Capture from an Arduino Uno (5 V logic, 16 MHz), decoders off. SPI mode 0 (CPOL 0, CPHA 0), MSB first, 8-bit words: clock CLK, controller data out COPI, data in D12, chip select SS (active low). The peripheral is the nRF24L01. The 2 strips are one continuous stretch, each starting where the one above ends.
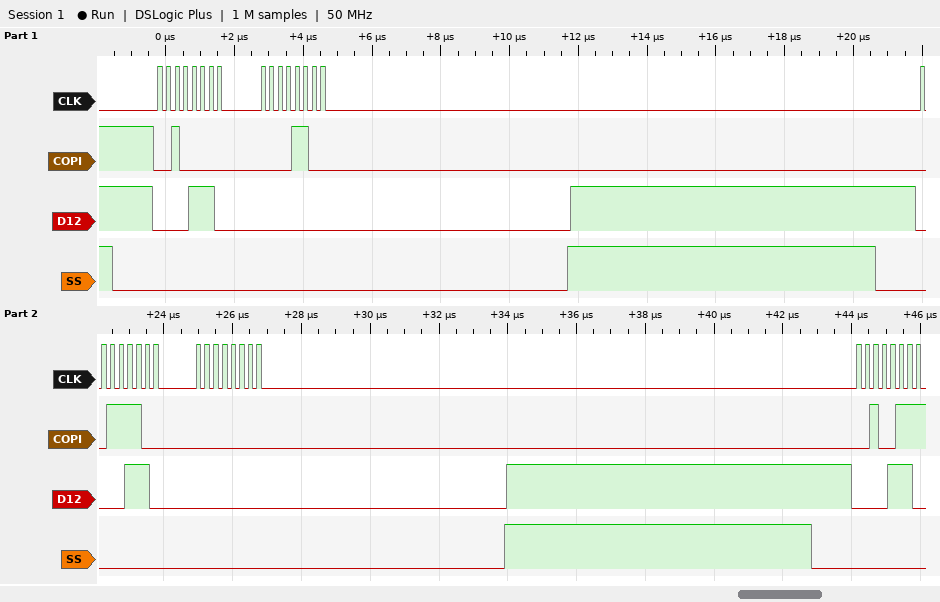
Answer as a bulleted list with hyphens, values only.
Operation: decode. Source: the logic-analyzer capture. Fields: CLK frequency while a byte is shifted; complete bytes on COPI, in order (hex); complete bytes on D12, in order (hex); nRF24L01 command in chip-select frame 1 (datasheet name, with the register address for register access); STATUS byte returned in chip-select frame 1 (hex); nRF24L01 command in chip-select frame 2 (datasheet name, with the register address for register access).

- 4 MHz
- 0x20 0x0C 0x3C 0x00 0x27
- 0x0E 0x00 0x0E 0x00 0x0E
- W_REGISTER 0x00
- 0x0E
- W_REGISTER 0x1C
